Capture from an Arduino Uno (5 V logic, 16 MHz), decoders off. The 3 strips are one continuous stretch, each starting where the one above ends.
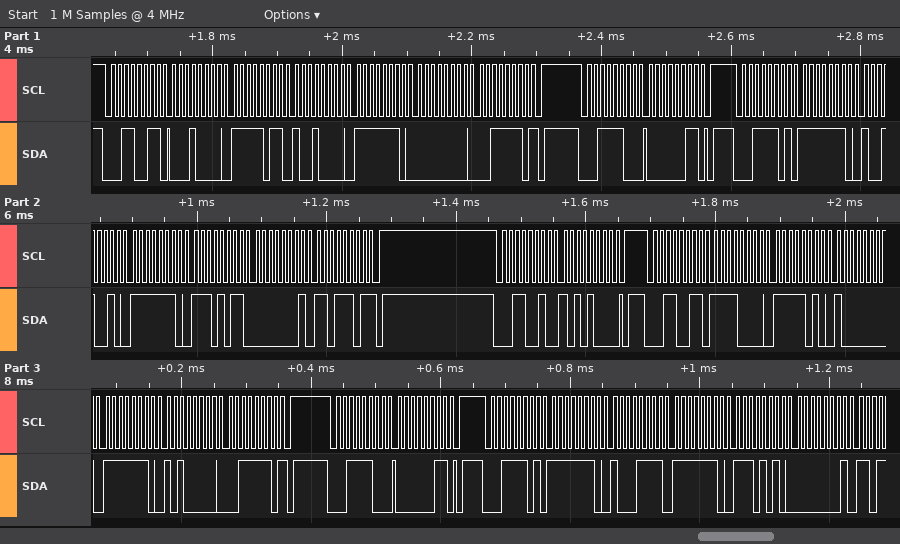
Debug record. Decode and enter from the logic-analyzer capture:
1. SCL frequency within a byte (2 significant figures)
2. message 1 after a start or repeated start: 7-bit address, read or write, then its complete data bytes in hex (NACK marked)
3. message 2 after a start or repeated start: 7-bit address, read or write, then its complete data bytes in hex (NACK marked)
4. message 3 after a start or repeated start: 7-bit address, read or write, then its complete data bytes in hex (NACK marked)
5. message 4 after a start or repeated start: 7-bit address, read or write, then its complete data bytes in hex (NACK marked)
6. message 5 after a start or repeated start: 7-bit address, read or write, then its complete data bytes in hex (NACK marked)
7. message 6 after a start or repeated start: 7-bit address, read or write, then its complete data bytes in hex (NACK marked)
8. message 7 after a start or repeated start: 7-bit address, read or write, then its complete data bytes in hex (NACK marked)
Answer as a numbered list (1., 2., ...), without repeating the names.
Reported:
1. 100 kHz
2. 0x19 read: 10 FB 90 FE 00 3E NACK
3. 0x1E write: 03
4. 0x1E read: FE 92 FE EB 01 DD NACK
5. 0x19 write: A8
6. 0x19 read: F0 FA 80 FE A0 3E NACK
7. 0x1E write: 03
8. 0x1E read: FE 8F FE EA 01
